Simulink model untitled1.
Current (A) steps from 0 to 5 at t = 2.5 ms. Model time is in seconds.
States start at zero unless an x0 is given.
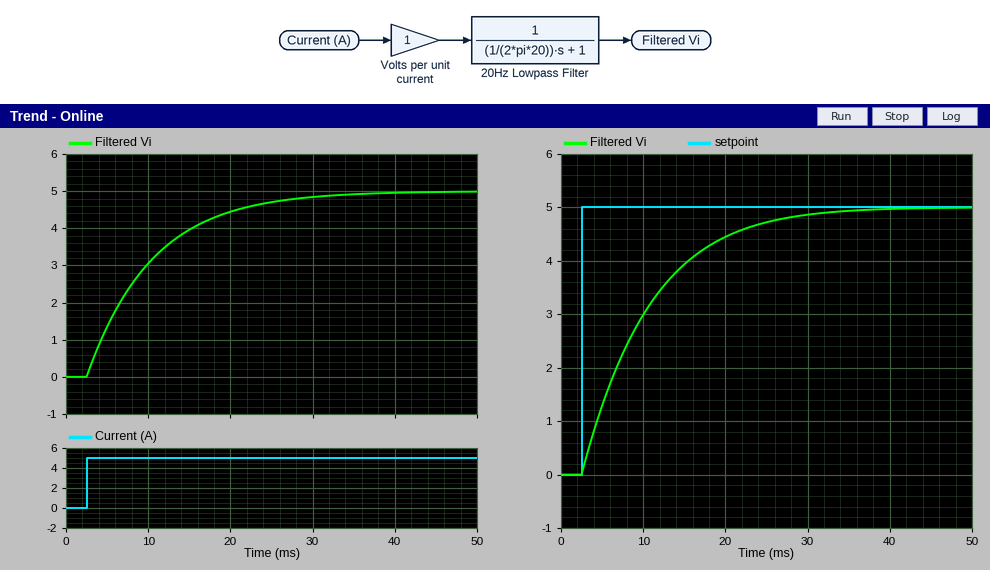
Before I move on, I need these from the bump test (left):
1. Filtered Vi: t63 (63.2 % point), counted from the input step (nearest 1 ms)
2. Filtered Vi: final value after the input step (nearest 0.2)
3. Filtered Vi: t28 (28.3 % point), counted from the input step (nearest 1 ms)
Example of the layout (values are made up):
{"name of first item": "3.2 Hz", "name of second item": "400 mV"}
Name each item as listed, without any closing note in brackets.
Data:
{"Filtered Vi: t63 (63.2 % point), counted from the input step": "8 ms", "Filtered Vi: final value after the input step": "5.0", "Filtered Vi: t28 (28.3 % point), counted from the input step": "3 ms"}
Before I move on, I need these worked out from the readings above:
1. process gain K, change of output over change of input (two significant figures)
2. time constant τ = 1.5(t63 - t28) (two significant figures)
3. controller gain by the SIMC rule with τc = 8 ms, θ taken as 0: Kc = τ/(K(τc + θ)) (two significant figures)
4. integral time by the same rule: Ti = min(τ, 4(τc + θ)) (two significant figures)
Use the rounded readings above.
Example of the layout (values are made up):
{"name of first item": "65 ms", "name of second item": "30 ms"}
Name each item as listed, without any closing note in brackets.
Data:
{"process gain K, change of output over change of input": "1.0", "time constant τ = 1.5(t63 - t28)": "7.5 ms", "controller gain by the SIMC rule with τc = 8 ms, θ taken as 0: Kc = τ/(K(τc + θ))": "0.94", "integral time by the same rule: Ti = min(τ, 4(τc + θ))": "7.5 ms"}
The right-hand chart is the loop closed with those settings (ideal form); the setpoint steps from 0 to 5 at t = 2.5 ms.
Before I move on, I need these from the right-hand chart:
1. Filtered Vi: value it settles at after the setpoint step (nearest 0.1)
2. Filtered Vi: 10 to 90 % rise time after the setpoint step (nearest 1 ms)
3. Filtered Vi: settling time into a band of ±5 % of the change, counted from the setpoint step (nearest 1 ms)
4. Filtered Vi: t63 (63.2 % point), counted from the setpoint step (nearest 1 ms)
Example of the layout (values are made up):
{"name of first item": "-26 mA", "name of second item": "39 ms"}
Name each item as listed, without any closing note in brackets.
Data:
{"Filtered Vi: value it settles at after the setpoint step": "5.0", "Filtered Vi: 10 to 90 % rise time after the setpoint step": "17 ms", "Filtered Vi: settling time into a band of ±5 % of the change, counted from the setpoint step": "23 ms", "Filtered Vi: t63 (63.2 % point), counted from the setpoint step": "8 ms"}
